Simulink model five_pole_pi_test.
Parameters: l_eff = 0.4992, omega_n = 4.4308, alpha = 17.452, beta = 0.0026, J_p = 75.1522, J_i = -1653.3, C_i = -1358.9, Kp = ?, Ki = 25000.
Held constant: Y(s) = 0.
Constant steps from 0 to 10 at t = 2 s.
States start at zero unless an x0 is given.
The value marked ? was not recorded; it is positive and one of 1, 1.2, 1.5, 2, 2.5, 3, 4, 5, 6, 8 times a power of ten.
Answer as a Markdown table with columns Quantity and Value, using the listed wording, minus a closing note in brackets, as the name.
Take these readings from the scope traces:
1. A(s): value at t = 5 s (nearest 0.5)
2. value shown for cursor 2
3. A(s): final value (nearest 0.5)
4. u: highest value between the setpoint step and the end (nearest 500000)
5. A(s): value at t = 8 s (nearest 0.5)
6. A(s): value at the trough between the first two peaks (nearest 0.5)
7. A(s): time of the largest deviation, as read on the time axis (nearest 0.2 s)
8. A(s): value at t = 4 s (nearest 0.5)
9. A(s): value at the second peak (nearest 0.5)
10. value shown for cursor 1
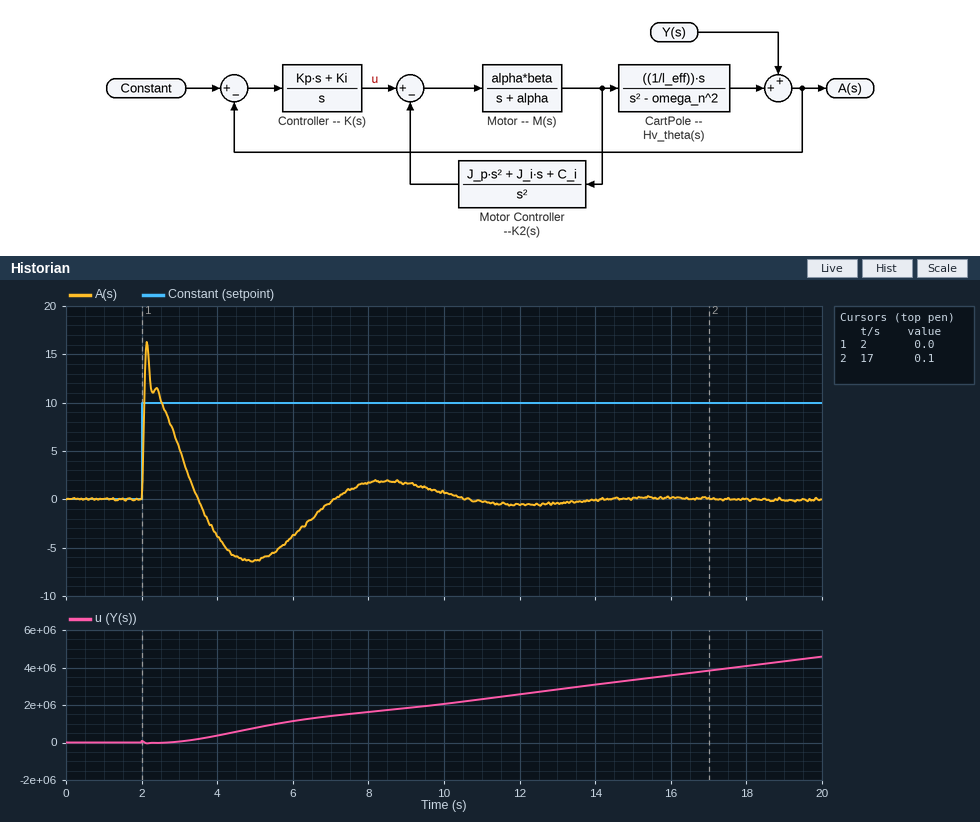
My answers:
| Quantity | Value |
|---|---|
| A(s): value at t = 5 s | -6.5 |
| value shown for cursor 2 | 0.1 |
| A(s): final value | 0.0 |
| u: highest value between the setpoint step and the end | 4500000 |
| A(s): value at t = 8 s | 1.5 |
| A(s): value at the trough between the first two peaks | -6.5 |
| A(s): time of the largest deviation, as read on the time axis | 2.2 s |
| A(s): value at t = 4 s | -4.0 |
| A(s): value at the second peak | 2.0 |
| value shown for cursor 1 | 0.0 |
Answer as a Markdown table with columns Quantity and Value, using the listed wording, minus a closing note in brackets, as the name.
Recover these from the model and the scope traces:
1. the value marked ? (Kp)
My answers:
| Quantity | Value |
|---|---|
| the value marked ? | 8000 |
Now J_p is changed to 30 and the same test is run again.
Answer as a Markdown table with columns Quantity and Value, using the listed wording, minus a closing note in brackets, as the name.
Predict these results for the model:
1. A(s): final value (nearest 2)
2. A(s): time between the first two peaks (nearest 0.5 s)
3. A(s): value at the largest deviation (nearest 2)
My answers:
| Quantity | Value |
|---|---|
| A(s): final value | 0 |
| A(s): time between the first two peaks | 6.5 s |
| A(s): value at the largest deviation | 16 |
